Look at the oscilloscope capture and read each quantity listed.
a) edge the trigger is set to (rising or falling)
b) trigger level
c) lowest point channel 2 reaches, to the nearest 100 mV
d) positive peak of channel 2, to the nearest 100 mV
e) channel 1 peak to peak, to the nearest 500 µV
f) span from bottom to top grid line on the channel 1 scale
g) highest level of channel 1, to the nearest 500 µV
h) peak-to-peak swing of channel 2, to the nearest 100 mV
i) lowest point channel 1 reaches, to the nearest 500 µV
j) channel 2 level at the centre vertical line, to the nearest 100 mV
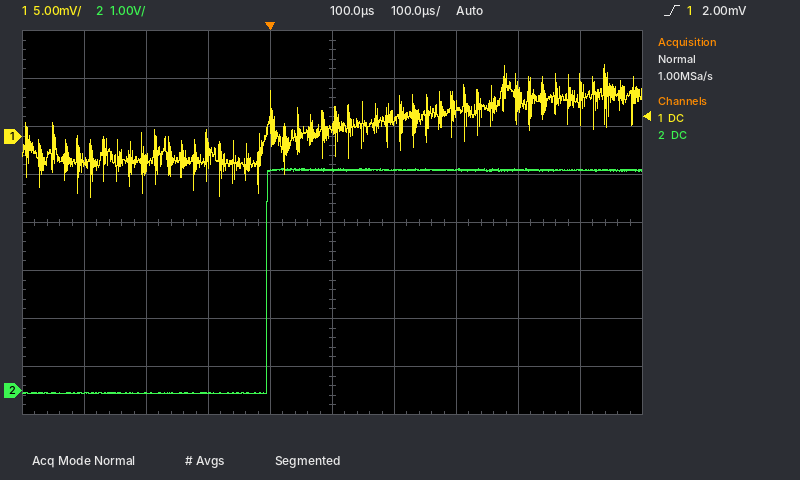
rising
2.00 mV
-100 mV
4.6 V
14.0 mV
40 mV
7.5 mV
4.7 V
-6.5 mV
4.6 V
